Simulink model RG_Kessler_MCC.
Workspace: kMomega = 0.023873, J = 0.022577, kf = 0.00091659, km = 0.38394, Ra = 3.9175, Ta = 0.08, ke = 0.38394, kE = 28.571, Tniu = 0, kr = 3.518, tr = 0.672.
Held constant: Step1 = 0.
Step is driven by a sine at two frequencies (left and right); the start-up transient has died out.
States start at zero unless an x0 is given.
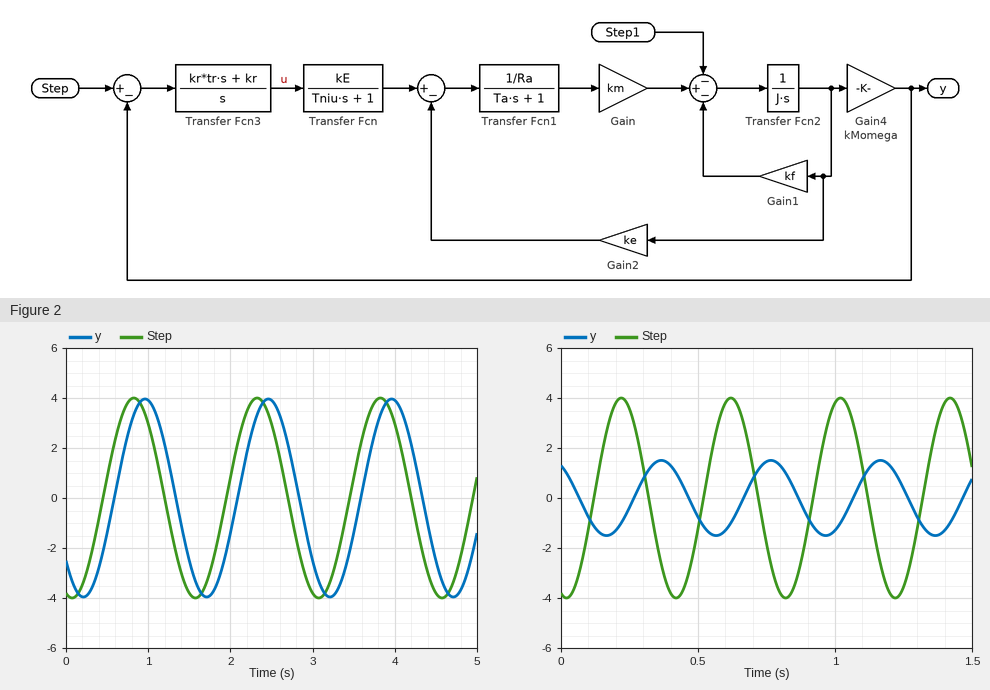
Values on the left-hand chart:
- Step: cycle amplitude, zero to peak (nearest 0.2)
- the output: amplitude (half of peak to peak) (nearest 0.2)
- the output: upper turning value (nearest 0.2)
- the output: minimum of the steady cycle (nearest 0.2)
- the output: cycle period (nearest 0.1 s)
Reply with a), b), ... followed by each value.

a) 4.0
b) 4.0
c) 4.0
d) -4.0
e) 1.5 s
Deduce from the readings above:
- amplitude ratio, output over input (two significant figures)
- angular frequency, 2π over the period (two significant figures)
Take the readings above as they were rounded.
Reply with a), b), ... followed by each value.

a) 1.0
b) 4.2 rad/s
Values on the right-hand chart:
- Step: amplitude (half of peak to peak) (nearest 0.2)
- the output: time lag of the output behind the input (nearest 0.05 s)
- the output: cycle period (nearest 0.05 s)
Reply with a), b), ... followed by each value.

a) 4.0
b) 0.15 s
c) 0.40 s
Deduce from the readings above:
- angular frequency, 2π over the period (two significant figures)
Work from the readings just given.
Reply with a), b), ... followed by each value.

a) 16 rad/s
